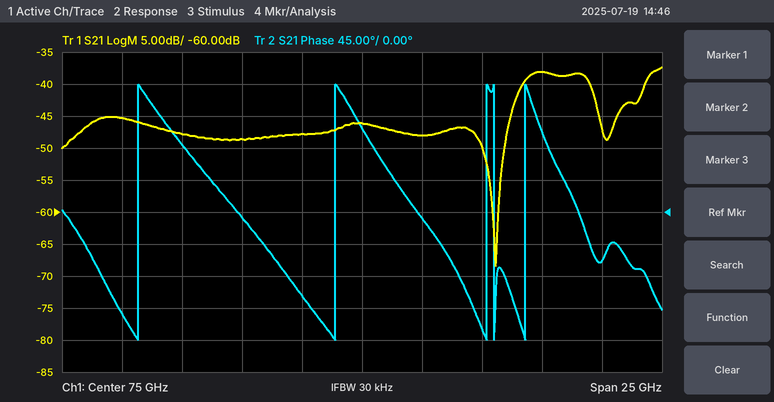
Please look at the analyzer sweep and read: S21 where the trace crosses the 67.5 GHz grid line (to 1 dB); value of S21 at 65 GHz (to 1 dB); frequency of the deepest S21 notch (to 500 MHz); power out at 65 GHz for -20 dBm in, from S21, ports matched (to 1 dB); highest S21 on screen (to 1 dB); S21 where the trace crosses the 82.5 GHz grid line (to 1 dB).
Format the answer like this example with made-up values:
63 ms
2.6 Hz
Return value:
-48 dB
-45 dB
80.5 GHz
-65 dBm
-37 dB
-38 dB
